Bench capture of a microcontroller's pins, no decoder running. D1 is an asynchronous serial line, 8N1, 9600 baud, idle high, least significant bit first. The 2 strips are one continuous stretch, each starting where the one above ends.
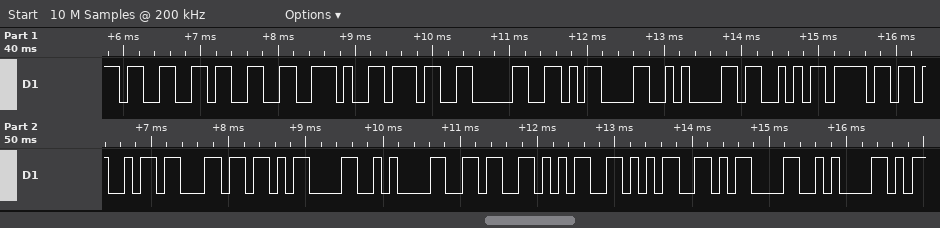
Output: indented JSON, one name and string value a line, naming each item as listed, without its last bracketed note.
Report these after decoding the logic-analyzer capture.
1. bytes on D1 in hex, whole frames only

{
  "bytes on D1 in hex, whole frames only": "0x33 0x33 0x2E 0x37 0x30 0x0D 0x0A 0x53 0x6F 0x69 0x6C 0x0D 0x0A 0x36 0x35 0x35 0x0D 0x0A"
}
